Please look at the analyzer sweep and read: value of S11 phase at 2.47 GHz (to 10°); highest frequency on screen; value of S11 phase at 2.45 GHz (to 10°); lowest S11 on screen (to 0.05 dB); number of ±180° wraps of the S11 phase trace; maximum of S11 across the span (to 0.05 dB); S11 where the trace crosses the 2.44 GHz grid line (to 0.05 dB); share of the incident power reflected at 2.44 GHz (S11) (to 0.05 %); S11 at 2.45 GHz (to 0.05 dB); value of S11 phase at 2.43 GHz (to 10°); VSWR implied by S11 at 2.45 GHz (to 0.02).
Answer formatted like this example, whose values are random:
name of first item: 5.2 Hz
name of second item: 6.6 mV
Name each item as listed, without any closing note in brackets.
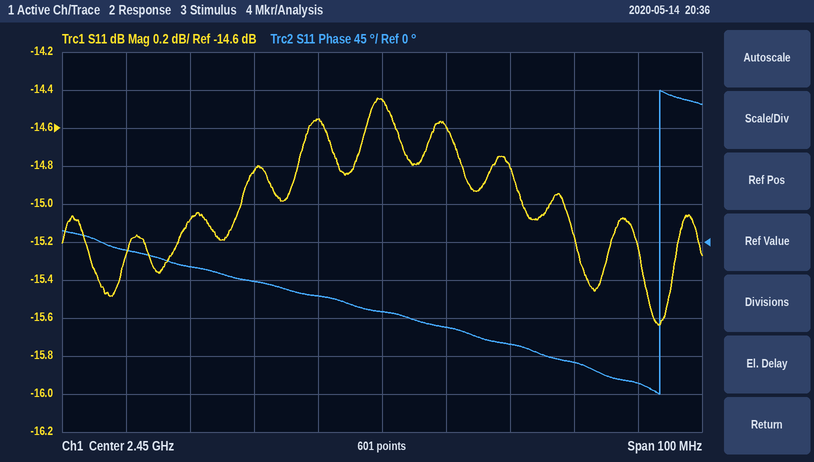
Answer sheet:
value of S11 phase at 2.47 GHz: -120°
highest frequency on screen: 2.5 GHz
value of S11 phase at 2.45 GHz: -80°
lowest S11 on screen: -15.65 dB
number of ±180° wraps of the S11 phase trace: 1
maximum of S11 across the span: -14.45 dB
S11 where the trace crosses the 2.44 GHz grid line: -14.55 dB
share of the incident power reflected at 2.44 GHz (S11): 3.50 %
S11 at 2.45 GHz: -14.45 dB
value of S11 phase at 2.43 GHz: -50°
VSWR implied by S11 at 2.45 GHz: 1.46
